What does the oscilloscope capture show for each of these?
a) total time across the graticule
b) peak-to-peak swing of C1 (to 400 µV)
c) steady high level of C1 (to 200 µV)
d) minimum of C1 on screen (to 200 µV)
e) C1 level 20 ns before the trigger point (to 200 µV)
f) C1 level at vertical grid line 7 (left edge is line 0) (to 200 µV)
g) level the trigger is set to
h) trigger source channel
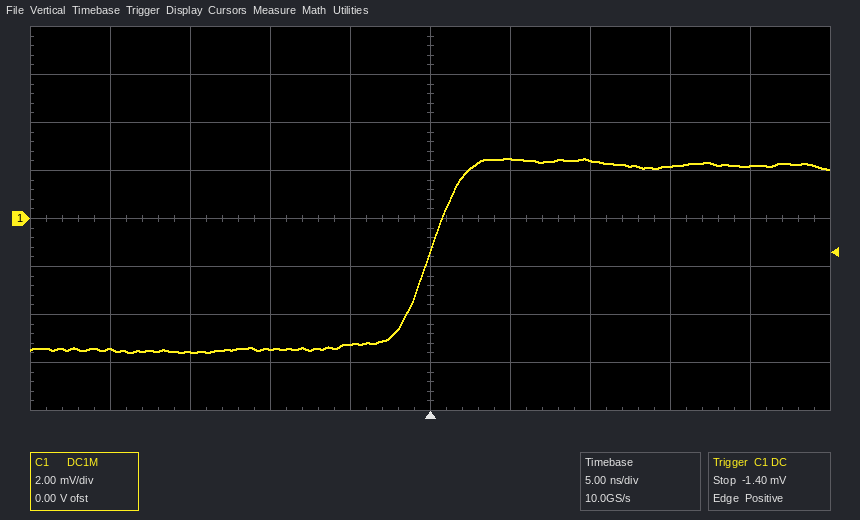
50 ns
8.0 mV
2.2 mV
-5.6 mV
-5.4 mV
2.4 mV
-1.40 mV
C1
